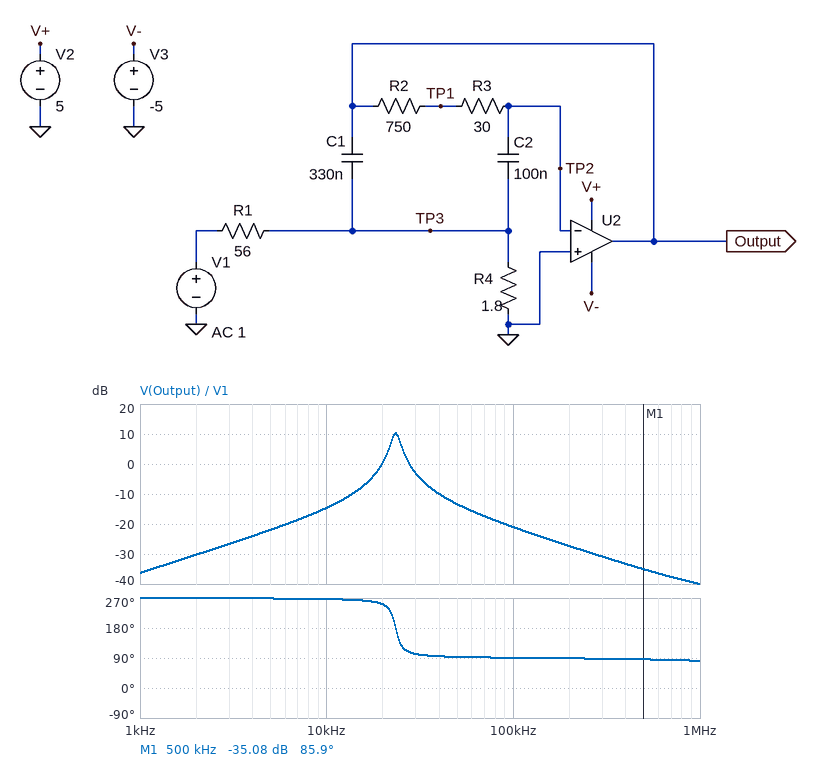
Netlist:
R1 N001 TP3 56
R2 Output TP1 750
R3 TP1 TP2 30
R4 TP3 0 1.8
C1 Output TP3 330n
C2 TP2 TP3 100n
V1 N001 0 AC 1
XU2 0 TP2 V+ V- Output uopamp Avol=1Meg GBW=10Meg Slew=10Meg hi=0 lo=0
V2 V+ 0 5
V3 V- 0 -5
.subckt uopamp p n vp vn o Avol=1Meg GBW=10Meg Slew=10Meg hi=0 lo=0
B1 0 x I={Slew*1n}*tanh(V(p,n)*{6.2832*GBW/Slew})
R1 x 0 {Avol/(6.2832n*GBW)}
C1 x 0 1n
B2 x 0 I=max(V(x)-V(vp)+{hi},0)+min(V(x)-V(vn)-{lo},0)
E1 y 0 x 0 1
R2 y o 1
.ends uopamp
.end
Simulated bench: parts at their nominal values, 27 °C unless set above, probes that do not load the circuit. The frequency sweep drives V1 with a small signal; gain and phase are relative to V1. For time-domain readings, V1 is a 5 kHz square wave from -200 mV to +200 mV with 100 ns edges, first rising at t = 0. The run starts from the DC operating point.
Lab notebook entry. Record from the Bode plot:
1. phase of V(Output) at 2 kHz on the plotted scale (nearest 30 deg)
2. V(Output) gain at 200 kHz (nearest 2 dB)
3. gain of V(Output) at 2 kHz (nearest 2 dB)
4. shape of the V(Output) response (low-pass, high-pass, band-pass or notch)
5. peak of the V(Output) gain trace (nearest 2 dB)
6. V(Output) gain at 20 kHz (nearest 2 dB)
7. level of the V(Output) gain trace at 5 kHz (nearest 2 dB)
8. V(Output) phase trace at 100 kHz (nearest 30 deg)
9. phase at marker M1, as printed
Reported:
270 deg
-28 dB
-30 dB
band-pass
10 dB
0 dB
-22 dB
90 deg
85.9 deg
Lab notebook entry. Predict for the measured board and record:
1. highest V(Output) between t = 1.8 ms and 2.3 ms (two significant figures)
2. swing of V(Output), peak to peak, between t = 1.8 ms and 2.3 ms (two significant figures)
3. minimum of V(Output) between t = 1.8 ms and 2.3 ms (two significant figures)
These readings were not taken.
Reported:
150 mV
300 mV
-150 mV
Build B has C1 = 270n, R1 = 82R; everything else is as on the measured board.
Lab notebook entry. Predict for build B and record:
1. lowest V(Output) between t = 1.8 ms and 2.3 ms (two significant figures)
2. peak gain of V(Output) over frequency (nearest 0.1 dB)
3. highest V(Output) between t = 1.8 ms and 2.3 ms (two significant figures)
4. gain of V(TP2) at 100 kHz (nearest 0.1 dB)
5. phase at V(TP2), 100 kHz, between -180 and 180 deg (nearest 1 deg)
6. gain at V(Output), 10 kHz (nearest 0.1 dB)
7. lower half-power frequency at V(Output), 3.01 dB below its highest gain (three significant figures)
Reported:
-160 mV
8.3 dB
160 mV
-62.4 dB
10 deg
-18.1 dB
24.4 kHz
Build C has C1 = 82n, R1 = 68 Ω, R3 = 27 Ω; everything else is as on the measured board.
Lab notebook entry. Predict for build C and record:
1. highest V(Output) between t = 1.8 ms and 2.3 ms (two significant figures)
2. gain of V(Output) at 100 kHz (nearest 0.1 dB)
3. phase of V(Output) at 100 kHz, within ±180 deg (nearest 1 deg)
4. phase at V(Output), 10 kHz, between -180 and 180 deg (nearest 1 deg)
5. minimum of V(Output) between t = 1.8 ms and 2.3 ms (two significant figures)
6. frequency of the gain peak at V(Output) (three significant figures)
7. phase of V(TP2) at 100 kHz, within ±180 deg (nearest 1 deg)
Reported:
300 mV
-9.8 dB
92 deg
-91 deg
-300 mV
45.2 kHz
5 deg
